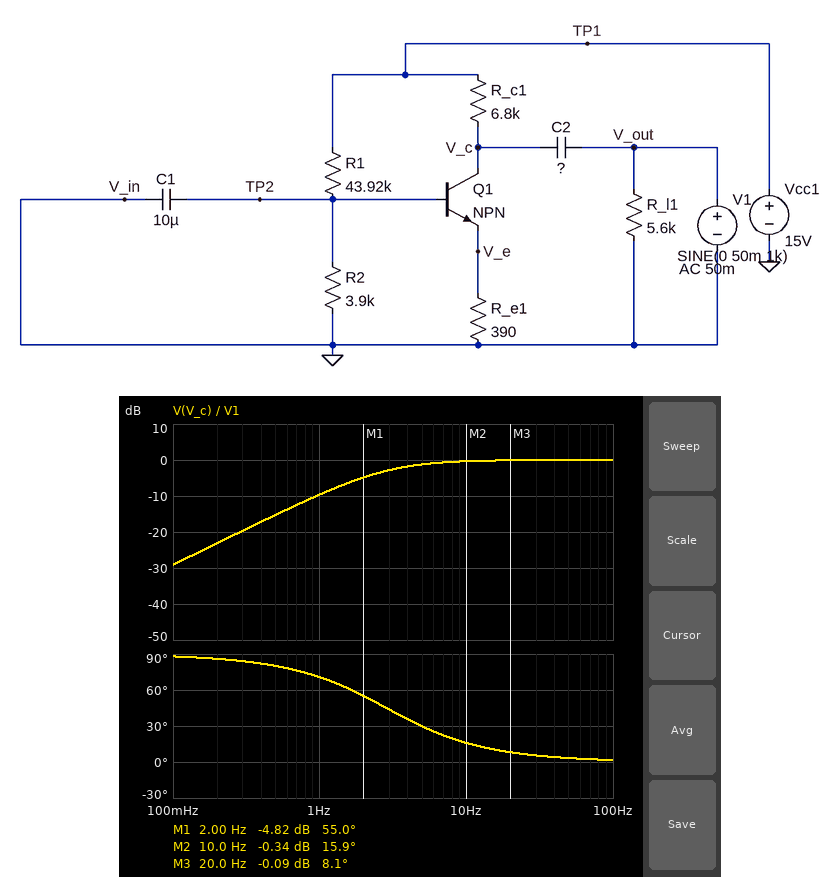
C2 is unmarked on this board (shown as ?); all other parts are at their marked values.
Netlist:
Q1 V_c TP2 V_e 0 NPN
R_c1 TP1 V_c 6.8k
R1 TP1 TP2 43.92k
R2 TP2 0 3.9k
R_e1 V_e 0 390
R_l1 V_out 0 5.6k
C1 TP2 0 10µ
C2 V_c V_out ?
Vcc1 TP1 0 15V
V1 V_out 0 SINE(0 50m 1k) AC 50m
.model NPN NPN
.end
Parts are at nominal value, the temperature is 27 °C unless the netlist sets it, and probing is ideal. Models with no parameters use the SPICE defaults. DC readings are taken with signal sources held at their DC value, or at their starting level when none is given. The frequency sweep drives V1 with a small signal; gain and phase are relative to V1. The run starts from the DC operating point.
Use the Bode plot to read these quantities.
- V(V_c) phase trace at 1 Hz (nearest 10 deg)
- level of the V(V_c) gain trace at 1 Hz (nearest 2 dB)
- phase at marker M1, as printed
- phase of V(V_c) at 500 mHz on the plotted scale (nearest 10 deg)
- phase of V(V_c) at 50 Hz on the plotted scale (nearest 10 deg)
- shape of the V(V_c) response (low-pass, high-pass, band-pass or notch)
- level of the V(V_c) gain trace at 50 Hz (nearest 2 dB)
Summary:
70 deg
-10 dB
55.0 deg
80 deg
0 deg
high-pass
0 dB
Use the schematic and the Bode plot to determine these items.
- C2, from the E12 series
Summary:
8.2 µF
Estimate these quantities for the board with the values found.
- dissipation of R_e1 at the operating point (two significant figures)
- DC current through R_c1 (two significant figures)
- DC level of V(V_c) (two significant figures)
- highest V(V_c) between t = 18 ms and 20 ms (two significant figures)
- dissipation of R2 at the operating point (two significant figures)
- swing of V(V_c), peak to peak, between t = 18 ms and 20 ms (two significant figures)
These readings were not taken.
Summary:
430 µW
1.0 mA
7.9 V
8.0 V
360 µW
100 mV
